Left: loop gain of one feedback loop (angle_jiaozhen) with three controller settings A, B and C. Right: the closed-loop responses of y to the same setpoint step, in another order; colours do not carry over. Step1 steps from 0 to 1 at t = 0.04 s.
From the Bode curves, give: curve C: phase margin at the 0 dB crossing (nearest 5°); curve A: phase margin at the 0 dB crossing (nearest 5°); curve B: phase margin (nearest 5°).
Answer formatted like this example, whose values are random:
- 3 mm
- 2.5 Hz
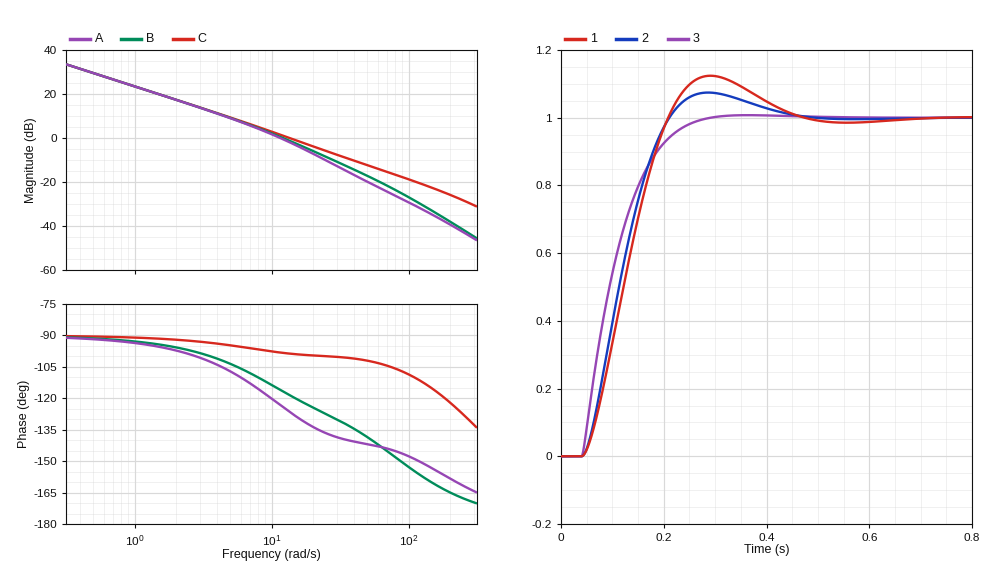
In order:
- 80°
- 55°
- 65°
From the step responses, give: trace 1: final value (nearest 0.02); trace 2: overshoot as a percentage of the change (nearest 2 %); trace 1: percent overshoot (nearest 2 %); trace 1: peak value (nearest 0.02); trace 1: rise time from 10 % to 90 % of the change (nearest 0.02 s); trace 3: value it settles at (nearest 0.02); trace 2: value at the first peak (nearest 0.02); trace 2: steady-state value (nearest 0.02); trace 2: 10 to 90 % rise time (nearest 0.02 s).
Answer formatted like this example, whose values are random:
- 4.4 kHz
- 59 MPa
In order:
- 1.00
- 8 %
- 12 %
- 1.12
- 0.12 s
- 1.00
- 1.08
- 1.00
- 0.12 s
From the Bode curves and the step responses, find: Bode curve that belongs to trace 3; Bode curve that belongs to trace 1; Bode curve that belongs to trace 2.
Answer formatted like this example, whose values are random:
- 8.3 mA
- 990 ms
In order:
- C
- A
- B
